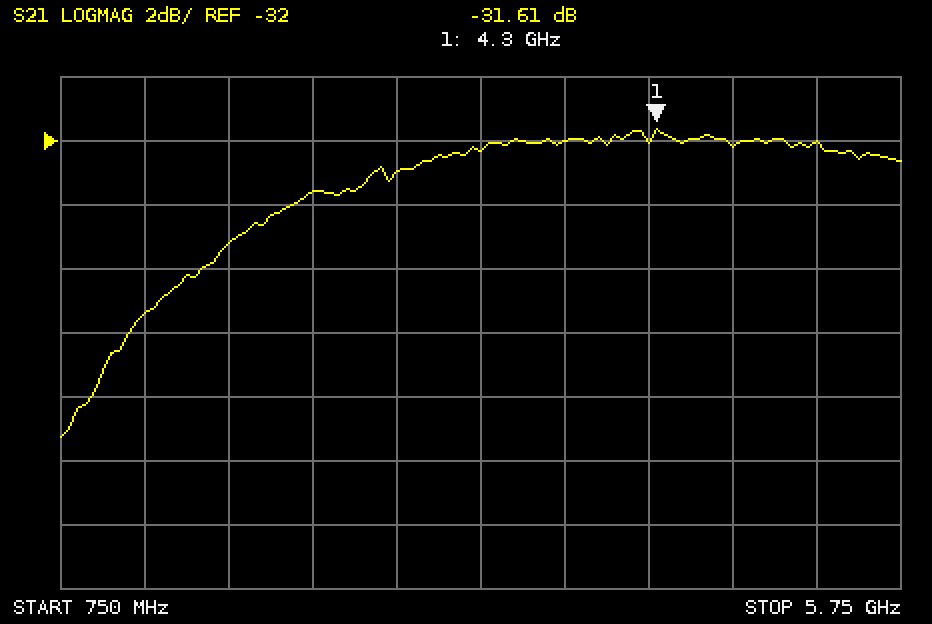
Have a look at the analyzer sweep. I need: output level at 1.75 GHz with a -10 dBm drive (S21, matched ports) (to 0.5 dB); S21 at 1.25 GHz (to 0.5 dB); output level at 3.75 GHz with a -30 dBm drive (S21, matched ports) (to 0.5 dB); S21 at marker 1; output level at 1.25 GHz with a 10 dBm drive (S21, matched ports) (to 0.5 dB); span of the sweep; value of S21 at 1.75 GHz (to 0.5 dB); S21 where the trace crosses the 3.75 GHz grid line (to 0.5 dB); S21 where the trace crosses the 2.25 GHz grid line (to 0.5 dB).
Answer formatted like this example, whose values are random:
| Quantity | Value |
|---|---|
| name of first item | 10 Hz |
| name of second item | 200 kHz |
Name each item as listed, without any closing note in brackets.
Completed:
| Quantity | Value |
|---|---|
| output level at 1.75 GHz with a -10 dBm drive (S21, matched ports) | -45.0 dBm |
| S21 at 1.25 GHz | -37.5 dB |
| output level at 3.75 GHz with a -30 dBm drive (S21, matched ports) | -62.0 dBm |
| S21 at marker 1 | -31.61 dB |
| output level at 1.25 GHz with a 10 dBm drive (S21, matched ports) | -27.5 dBm |
| span of the sweep | 5 GHz |
| value of S21 at 1.75 GHz | -35.0 dB |
| S21 where the trace crosses the 3.75 GHz grid line | -32.0 dB |
| S21 where the trace crosses the 2.25 GHz grid line | -33.5 dB |
